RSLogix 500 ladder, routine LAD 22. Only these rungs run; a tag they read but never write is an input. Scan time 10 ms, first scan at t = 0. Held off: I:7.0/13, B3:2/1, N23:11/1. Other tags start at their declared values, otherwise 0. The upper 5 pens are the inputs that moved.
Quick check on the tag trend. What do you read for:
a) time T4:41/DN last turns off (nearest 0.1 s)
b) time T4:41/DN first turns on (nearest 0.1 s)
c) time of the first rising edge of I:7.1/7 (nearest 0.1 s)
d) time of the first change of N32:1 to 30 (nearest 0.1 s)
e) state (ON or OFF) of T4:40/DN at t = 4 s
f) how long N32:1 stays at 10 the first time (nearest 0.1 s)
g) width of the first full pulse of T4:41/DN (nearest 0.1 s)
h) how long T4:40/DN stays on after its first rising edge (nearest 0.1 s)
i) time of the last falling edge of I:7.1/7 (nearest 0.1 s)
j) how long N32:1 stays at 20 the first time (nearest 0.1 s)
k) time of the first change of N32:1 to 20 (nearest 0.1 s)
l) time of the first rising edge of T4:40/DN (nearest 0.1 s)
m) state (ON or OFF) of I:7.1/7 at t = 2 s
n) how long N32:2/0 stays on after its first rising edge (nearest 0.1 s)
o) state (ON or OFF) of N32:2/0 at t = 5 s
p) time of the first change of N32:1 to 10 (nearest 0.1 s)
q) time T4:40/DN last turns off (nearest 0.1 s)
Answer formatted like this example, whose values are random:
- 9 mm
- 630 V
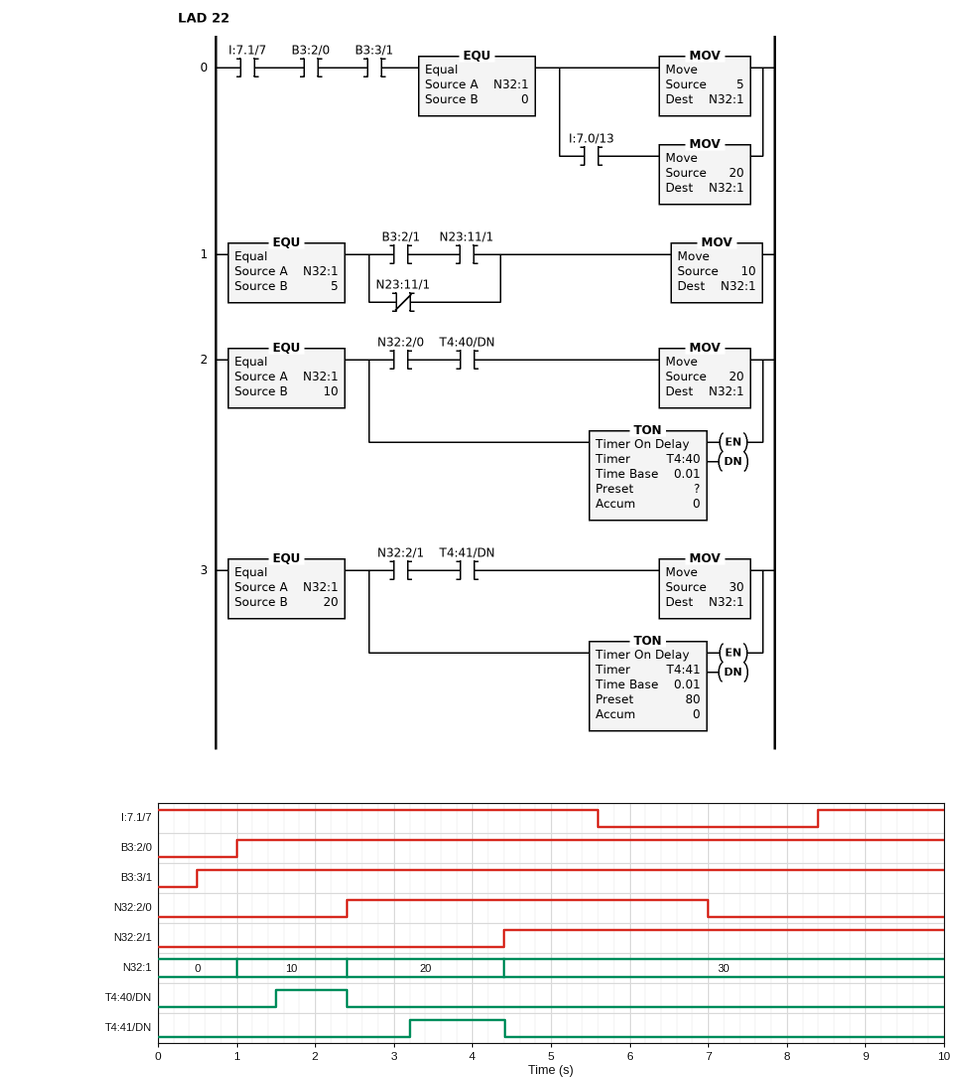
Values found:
- 4.4 s
- 3.2 s
- 8.4 s
- 4.4 s
- OFF
- 1.4 s
- 1.2 s
- 0.9 s
- 5.6 s
- 2.0 s
- 2.4 s
- 1.5 s
- ON
- 4.6 s
- ON
- 1.0 s
- 2.4 s
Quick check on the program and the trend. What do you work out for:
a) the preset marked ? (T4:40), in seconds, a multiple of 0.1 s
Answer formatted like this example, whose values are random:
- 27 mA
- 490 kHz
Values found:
- 0.5 s
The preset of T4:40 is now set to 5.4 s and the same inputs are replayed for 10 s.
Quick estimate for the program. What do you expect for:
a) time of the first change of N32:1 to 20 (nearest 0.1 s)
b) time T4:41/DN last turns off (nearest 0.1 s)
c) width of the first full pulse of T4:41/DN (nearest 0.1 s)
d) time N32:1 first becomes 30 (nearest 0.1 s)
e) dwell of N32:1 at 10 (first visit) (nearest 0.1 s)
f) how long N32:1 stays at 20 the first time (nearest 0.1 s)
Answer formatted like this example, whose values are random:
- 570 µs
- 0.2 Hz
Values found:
- 6.4 s
- 7.2 s
- 0.0 s
- 7.2 s
- 5.4 s
- 0.8 s
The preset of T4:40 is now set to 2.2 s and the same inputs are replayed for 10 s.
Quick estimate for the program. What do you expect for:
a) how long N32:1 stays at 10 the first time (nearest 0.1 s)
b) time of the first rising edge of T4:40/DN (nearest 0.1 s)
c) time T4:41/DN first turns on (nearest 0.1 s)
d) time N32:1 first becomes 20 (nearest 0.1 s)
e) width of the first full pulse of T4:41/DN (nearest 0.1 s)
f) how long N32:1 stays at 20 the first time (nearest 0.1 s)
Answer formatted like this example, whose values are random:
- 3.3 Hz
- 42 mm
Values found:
- 2.2 s
- 3.2 s
- 4.0 s
- 3.2 s
- 0.4 s
- 1.2 s
